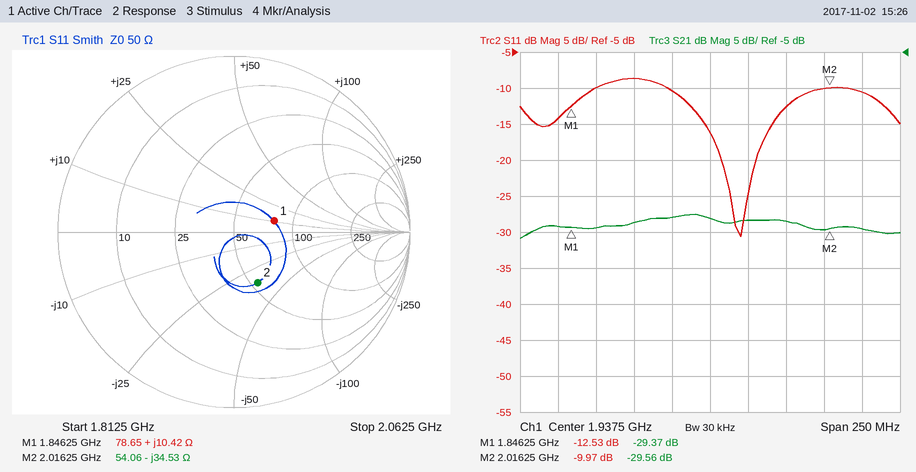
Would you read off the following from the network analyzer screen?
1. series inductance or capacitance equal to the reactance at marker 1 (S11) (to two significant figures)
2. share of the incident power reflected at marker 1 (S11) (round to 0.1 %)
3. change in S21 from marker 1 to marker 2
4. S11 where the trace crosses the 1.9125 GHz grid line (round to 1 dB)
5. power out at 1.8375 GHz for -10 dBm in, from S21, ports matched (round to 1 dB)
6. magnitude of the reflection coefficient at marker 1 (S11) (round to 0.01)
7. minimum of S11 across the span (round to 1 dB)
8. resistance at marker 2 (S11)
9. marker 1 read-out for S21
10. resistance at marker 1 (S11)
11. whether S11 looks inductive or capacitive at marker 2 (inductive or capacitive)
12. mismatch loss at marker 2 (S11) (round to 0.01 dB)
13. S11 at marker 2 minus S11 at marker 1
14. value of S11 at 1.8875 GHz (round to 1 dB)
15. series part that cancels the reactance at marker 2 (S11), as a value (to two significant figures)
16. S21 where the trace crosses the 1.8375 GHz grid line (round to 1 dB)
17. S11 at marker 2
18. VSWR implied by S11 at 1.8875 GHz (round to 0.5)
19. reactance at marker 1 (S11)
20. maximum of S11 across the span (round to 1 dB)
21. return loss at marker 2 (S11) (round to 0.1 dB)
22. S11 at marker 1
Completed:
900 pH
5.6 %
-0.19 dB
-10 dB
-39 dBm
0.24
-31 dB
54.06 Ω
-29.37 dB
78.65 Ω
capacitive
0.46 dB
2.56 dB
-9 dB
2.7 nH
-29 dB
-9.97 dB
2.0
+10.42 Ω
-9 dB
10.0 dB
-12.53 dB
